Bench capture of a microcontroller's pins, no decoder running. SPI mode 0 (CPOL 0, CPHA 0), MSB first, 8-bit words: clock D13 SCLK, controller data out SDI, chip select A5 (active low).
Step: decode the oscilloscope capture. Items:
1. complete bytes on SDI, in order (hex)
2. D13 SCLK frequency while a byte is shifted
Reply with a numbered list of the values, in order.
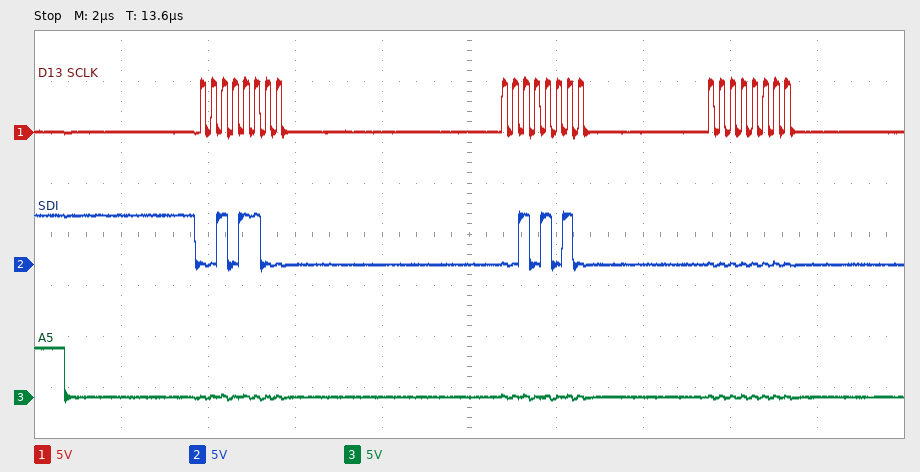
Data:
1. 2C 2A 00
2. 4 MHz
